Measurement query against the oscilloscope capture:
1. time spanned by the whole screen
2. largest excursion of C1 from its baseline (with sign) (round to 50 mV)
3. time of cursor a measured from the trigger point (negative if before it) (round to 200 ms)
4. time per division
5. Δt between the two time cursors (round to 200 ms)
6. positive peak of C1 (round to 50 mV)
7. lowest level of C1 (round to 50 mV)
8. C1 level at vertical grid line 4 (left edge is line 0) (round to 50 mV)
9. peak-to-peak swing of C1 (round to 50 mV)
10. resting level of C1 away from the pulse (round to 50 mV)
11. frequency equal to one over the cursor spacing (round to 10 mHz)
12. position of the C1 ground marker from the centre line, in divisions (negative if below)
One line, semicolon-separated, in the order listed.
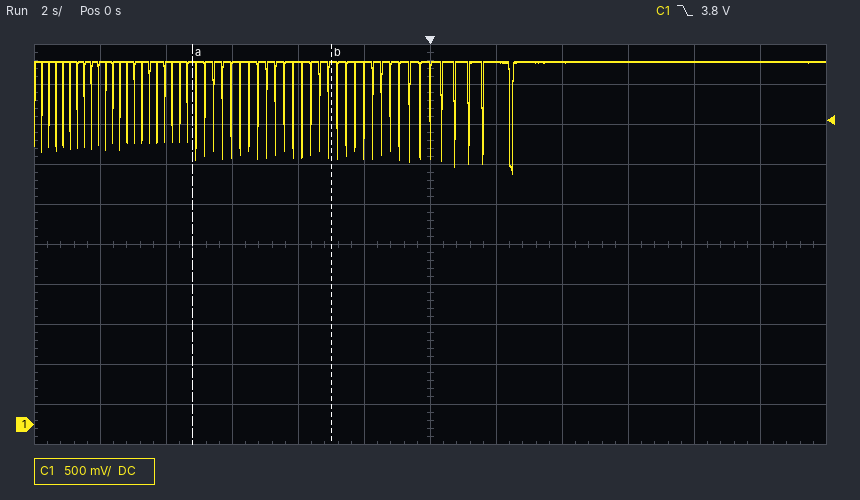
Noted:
24 s; -1.40 V; -7.2 s; 2 s; 4.2 s; 4.55 V; 3.15 V; 4.55 V; 1.40 V; 4.55 V; 240 mHz; -4.5 div
